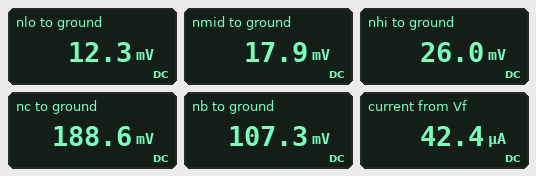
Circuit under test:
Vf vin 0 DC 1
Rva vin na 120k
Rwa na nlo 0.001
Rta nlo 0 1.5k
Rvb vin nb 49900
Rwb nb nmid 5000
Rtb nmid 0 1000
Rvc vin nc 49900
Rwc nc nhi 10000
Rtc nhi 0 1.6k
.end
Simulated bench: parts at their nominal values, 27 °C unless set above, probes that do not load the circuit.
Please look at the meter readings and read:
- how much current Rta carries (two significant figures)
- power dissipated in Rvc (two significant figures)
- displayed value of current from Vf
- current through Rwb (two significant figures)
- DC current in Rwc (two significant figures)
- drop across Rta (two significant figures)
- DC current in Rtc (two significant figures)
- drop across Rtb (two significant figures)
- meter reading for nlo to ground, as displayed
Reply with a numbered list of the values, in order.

1. 8.2 µA
2. 13 µW
3. 42.4 µA
4. 18 µA
5. 16 µA
6. 12 mV
7. 16 µA
8. 18 mV
9. 12.3 mV
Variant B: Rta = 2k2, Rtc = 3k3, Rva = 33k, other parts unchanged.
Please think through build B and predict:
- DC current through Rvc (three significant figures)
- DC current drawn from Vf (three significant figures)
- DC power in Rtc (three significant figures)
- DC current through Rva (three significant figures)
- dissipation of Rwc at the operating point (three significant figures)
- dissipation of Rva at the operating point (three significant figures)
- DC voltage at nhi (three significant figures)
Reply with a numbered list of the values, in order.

1. 15.8 µA
2. 62.1 µA
3. 826 nW
4. 28.4 µA
5. 2.50 µW
6. 26.6 µW
7. 52.2 mV
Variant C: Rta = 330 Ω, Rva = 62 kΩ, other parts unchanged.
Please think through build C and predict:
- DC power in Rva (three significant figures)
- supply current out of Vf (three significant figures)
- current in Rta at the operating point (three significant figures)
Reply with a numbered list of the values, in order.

1. 16.0 µW
2. 50.2 µA
3. 16.0 µA
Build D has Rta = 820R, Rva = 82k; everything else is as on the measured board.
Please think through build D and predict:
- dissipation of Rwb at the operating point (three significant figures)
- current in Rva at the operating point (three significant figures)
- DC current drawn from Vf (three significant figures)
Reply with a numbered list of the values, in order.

1. 1.60 µW
2. 12.1 µA
3. 46.2 µA
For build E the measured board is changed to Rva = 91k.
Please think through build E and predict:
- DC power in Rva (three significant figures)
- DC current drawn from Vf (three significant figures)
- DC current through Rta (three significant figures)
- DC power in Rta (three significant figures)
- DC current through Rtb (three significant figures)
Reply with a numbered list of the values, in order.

1. 10.6 µW
2. 45.0 µA
3. 10.8 µA
4. 175 nW
5. 17.9 µA
